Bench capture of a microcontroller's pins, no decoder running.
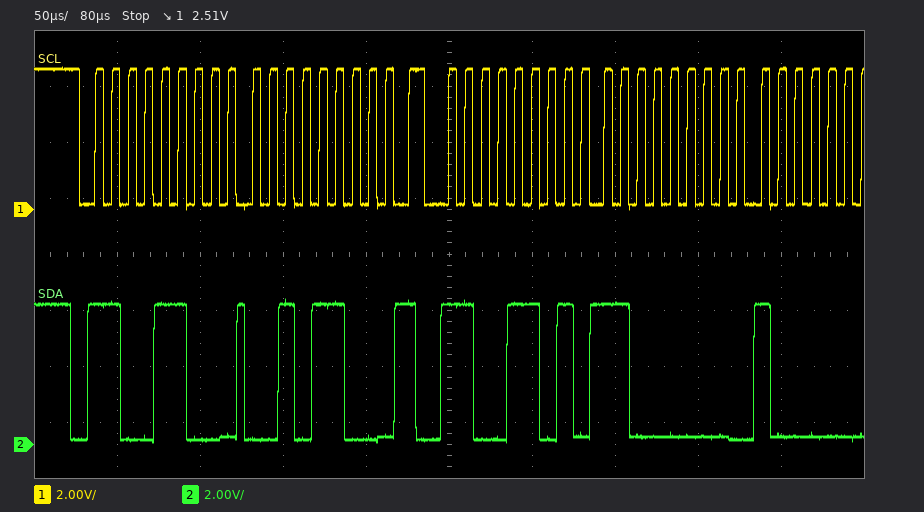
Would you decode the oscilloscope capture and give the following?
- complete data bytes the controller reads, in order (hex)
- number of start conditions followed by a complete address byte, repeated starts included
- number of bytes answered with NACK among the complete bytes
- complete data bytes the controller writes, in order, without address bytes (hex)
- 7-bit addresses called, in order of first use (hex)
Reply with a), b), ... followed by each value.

a) C0
b) 2
c) 0
d) 2C
e) 0x66
